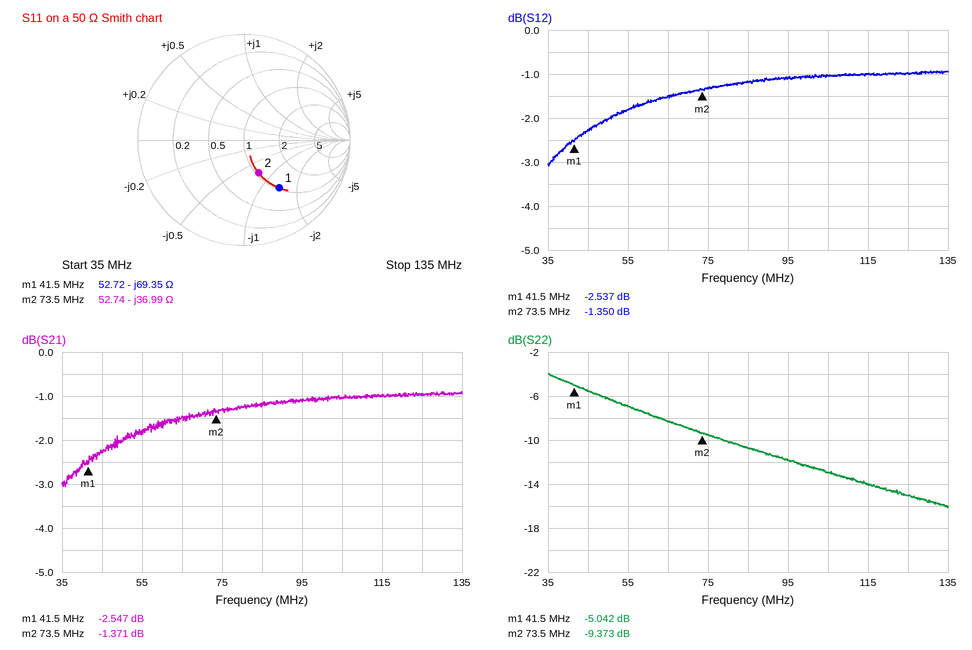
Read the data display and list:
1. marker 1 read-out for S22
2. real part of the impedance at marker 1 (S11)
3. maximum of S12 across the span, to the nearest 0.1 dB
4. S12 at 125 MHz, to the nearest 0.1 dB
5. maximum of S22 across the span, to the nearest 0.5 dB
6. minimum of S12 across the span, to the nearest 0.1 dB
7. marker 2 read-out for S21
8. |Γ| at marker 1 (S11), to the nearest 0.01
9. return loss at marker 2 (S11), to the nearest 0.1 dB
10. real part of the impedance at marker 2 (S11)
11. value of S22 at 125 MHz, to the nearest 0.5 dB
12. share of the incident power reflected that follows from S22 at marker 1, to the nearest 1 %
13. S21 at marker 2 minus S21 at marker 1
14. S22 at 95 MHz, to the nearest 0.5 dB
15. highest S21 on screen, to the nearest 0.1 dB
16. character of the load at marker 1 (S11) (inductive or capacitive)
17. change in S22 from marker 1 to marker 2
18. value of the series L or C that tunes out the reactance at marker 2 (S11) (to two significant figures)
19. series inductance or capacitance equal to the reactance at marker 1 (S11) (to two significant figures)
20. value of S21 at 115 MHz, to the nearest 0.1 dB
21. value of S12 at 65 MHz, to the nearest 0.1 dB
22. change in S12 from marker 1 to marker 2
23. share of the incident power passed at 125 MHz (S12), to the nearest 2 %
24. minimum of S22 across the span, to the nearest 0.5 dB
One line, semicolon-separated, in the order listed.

-5.042 dB; 52.72 Ω; -0.9 dB; -1.0 dB; -4.0 dB; -3.1 dB; -1.371 dB; 0.56; 9.4 dB; 52.74 Ω; -15.0 dB; 31 %; 1.176 dB; -12.0 dB; -0.9 dB; capacitive; -4.331 dB; 80 nH; 55 pF; -1.0 dB; -1.5 dB; 1.187 dB; 80 %; -16.0 dB
